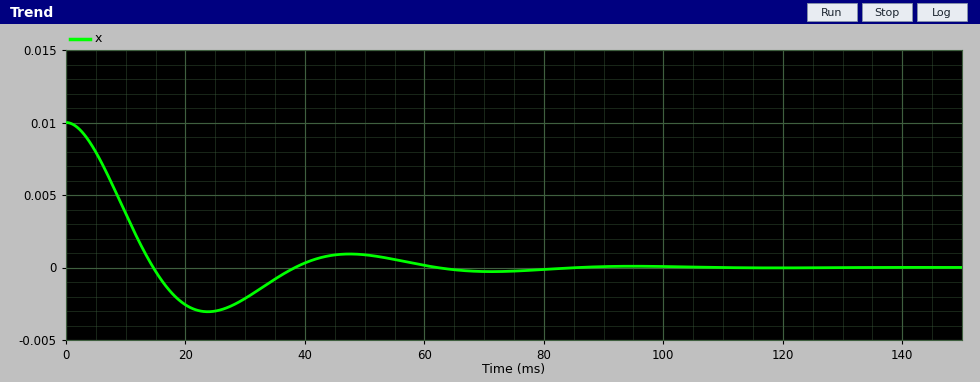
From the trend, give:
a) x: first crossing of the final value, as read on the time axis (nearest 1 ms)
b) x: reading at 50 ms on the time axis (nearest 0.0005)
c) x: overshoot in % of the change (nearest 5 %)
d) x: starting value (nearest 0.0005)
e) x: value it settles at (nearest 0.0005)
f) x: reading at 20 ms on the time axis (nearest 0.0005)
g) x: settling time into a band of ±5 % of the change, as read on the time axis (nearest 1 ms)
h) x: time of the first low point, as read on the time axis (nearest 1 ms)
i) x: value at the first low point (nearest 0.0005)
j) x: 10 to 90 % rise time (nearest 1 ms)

15 ms
0.0010
30 %
0.0100
0.0000
-0.0025
56 ms
24 ms
-0.0030
10 ms
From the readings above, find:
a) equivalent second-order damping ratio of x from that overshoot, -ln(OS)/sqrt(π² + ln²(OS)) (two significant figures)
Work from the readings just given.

0.36
